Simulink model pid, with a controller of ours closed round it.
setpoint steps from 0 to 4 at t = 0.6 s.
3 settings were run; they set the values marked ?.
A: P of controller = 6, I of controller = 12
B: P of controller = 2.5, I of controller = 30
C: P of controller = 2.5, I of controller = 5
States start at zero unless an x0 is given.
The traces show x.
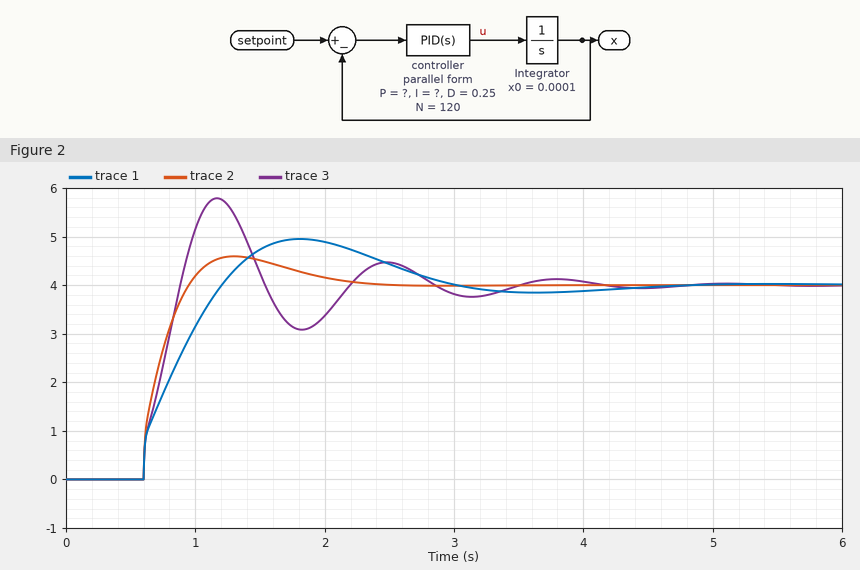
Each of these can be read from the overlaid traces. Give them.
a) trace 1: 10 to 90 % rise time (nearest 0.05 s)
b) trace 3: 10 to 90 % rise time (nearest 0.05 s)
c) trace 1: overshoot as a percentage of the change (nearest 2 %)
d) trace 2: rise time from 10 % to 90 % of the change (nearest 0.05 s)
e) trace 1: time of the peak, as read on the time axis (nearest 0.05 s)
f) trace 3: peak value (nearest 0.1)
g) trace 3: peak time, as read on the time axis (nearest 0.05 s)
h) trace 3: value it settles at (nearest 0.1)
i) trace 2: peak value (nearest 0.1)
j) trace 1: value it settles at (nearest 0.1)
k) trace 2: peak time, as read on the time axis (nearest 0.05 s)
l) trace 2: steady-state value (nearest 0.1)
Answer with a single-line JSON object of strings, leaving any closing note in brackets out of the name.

{"trace 1: 10 to 90 % rise time": "0.50 s", "trace 3: 10 to 90 % rise time": "0.25 s", "trace 1: overshoot as a percentage of the change": "24 %", "trace 2: rise time from 10 % to 90 % of the change": "0.25 s", "trace 1: time of the peak, as read on the time axis": "1.80 s", "trace 3: peak value": "5.8", "trace 3: peak time, as read on the time axis": "1.15 s", "trace 3: value it settles at": "4.0", "trace 2: peak value": "4.6", "trace 1: value it settles at": "4.0", "trace 2: peak time, as read on the time axis": "1.30 s", "trace 2: steady-state value": "4.0"}
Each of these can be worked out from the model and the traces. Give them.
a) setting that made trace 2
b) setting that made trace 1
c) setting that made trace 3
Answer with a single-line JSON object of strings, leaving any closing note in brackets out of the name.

{"setting that made trace 2": "A", "setting that made trace 1": "C", "setting that made trace 3": "B"}
